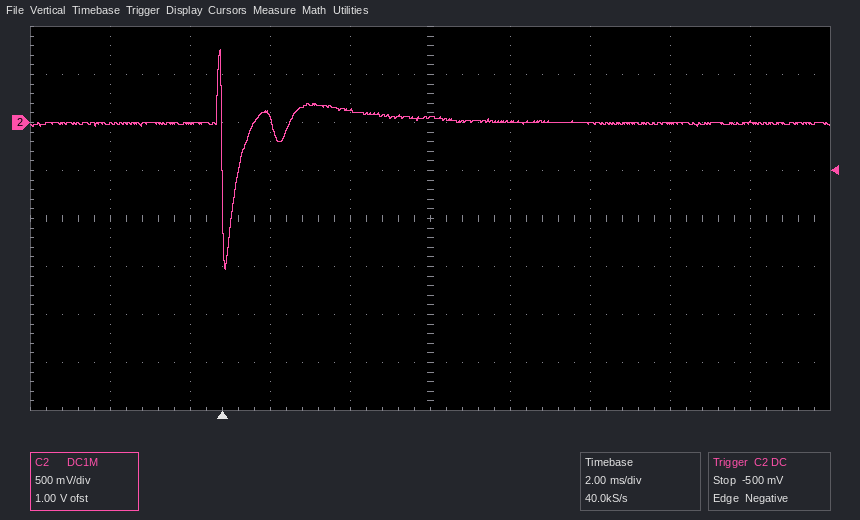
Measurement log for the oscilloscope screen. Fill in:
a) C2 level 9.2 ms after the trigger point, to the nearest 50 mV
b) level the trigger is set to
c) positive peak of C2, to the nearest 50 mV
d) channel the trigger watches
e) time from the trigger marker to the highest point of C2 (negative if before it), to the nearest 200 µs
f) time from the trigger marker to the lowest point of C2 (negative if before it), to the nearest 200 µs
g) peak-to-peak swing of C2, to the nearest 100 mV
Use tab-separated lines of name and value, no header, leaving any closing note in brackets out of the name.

C2 level 9.2 ms after the trigger point, to the nearest 50 mV	0 mV
level the trigger is set to	-500 mV
positive peak of C2, to the nearest 50 mV	750 mV
channel the trigger watches	C2
time from the trigger marker to the highest point of C2 (negative if before it), to the nearest 200 µs	0.0 ms
time from the trigger marker to the lowest point of C2 (negative if before it), to the nearest 200 µs	0.0 ms
peak-to-peak swing of C2, to the nearest 100 mV	2.30 V
